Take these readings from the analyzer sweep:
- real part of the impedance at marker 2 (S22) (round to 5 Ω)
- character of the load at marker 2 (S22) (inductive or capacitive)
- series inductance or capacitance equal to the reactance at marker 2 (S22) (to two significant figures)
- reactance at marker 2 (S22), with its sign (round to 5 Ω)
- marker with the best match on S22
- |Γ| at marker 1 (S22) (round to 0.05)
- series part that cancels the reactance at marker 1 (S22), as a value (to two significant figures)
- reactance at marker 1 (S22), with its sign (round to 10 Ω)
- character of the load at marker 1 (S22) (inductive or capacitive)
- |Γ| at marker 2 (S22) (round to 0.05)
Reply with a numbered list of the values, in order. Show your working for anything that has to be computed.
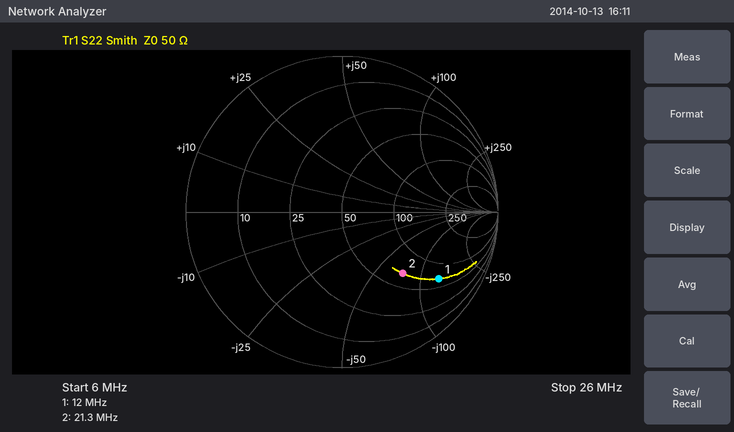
1. 65 Ω
2. capacitive
3. C = 1/(2π × 21.3 MHz × 75 Ω) ≈ 100 pF
4. -75 Ω
5. marker 2
6. 0.75
7. L = 130 Ω/(2π × 12 MHz) ≈ 1.7 µH
8. -130 Ω
9. capacitive
10. 0.55
